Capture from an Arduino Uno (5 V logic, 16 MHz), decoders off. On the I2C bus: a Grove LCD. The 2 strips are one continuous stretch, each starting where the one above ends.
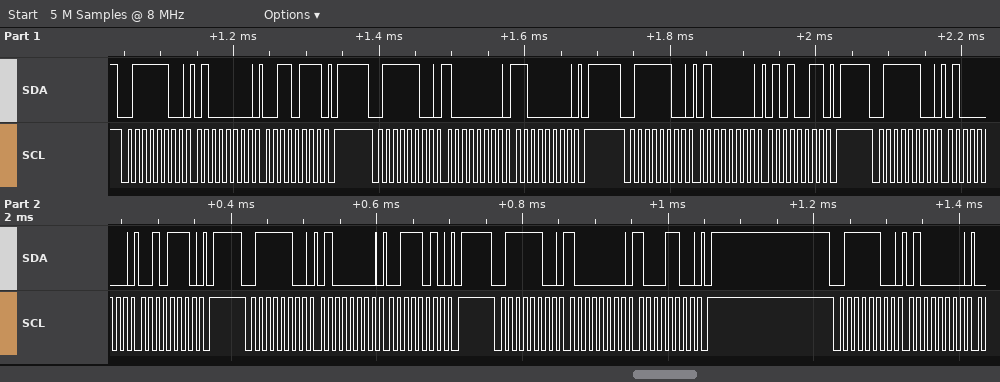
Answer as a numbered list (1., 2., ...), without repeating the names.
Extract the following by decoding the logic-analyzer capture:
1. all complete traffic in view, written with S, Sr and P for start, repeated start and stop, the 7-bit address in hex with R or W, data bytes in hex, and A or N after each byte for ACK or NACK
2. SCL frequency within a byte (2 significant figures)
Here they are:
1. S 3EW A 40 A 37 A P S 3EW A 80 A C0 A P S 3EW A 40 A 53 A P S 3EW A 40 A 2E A P S 3EW A 40 A 3A A P S 3EW A 80 A 8C A P S 3EW A 40 A
2. 100 kHz
